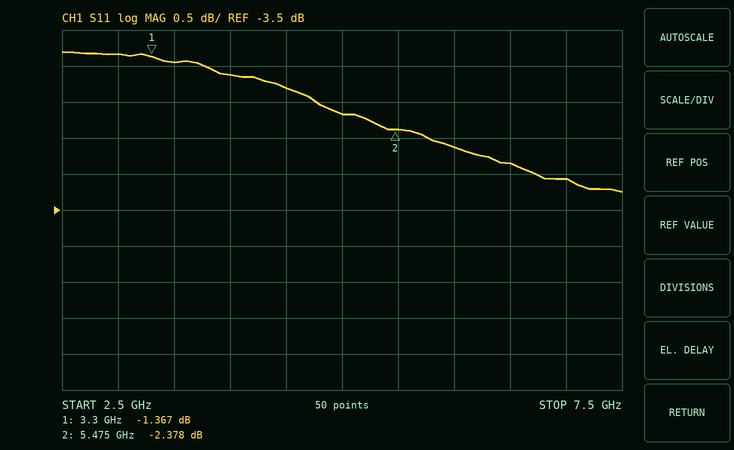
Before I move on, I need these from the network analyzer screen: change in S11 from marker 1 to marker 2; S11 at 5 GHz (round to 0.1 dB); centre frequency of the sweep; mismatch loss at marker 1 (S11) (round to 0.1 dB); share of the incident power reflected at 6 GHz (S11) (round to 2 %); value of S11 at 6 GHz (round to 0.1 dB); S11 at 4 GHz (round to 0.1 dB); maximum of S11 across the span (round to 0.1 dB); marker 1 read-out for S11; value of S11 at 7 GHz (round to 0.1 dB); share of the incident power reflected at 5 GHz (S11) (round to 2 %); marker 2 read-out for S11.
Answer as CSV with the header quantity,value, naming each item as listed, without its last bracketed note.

quantity,value
change in S11 from marker 1 to marker 2,-1.011 dB
S11 at 5 GHz,-2.2 dB
centre frequency of the sweep,5 GHz
mismatch loss at marker 1 (S11),5.7 dB
share of the incident power reflected at 6 GHz (S11),54 %
value of S11 at 6 GHz,-2.6 dB
S11 at 4 GHz,-1.6 dB
maximum of S11 across the span,-1.3 dB
marker 1 read-out for S11,-1.367 dB
value of S11 at 7 GHz,-3.1 dB
share of the incident power reflected at 5 GHz (S11),60 %
marker 2 read-out for S11,-2.378 dB
